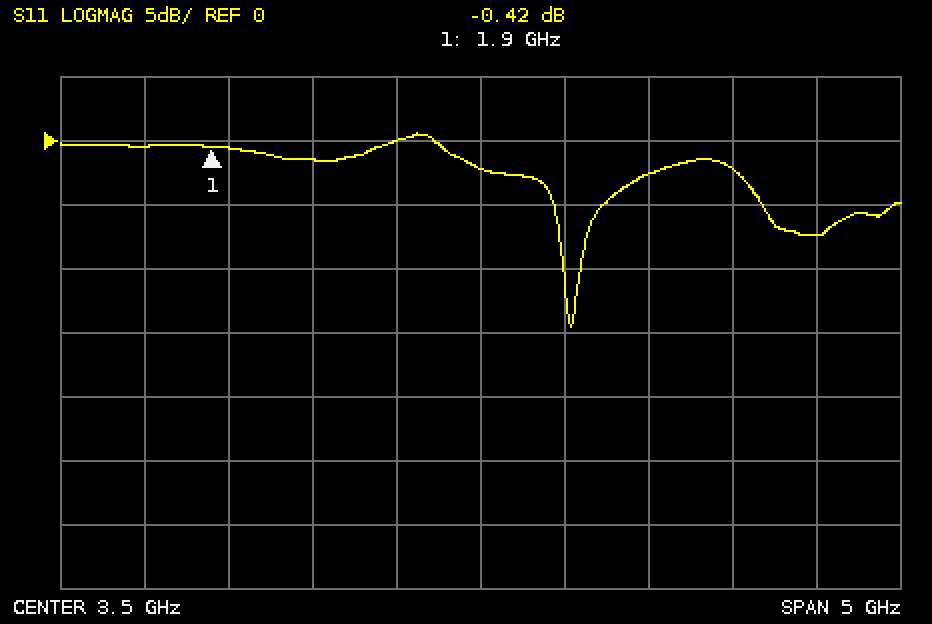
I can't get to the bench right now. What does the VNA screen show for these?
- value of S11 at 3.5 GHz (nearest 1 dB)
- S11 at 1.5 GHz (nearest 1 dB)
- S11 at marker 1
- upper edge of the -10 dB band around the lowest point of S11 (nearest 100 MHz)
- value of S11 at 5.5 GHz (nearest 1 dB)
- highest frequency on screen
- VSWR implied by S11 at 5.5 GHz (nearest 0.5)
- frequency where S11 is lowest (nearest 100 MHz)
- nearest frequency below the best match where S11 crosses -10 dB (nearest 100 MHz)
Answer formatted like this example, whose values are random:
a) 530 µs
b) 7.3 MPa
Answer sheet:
a) -2 dB
b) 0 dB
c) -0.42 dB
d) 4.1 GHz
e) -7 dB
f) 6 GHz
g) 2.5
h) 4.0 GHz
i) 4.0 GHz
